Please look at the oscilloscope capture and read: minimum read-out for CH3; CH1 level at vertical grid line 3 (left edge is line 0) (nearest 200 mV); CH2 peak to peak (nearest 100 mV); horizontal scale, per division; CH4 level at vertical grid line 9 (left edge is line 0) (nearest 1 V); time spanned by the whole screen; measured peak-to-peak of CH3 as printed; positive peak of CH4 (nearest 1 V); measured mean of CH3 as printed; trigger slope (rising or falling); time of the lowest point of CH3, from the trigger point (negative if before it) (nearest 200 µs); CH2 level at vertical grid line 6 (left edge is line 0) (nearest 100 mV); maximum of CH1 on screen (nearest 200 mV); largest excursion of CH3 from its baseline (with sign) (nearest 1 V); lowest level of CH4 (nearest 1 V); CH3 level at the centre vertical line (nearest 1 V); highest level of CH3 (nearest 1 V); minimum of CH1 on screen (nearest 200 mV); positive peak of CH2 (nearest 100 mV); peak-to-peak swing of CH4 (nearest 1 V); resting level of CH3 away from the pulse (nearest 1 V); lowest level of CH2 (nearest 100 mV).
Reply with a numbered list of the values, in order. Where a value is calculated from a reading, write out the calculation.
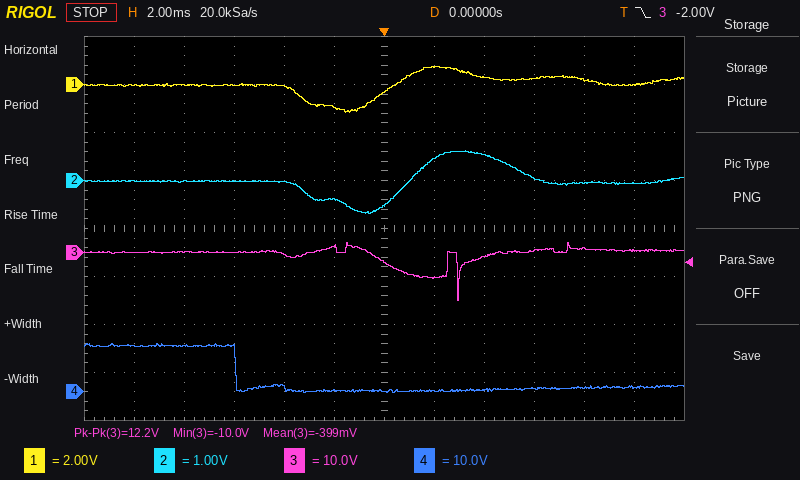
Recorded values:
1. -10.0 V
2. 0.0 V
3. 600 mV − (-700 mV) = 1.3 V
4. 2 ms
5. 1 V
6. 24 ms
7. 12.2 V
8. 10 V
9. -399 mV
10. falling
11. +3.0 ms
12. -500 mV
13. 800 mV
14. -10 V
15. 0 V
16. -2 V
17. 2 V
18. -1.2 V
19. 600 mV
20. 10 V − (0 V) = 10 V
21. 0 V
22. -700 mV
